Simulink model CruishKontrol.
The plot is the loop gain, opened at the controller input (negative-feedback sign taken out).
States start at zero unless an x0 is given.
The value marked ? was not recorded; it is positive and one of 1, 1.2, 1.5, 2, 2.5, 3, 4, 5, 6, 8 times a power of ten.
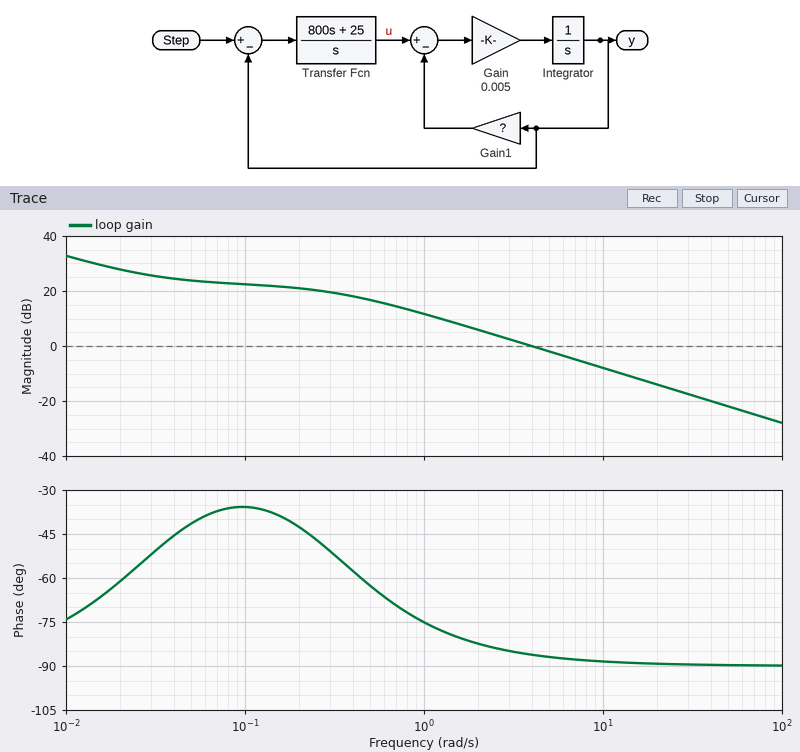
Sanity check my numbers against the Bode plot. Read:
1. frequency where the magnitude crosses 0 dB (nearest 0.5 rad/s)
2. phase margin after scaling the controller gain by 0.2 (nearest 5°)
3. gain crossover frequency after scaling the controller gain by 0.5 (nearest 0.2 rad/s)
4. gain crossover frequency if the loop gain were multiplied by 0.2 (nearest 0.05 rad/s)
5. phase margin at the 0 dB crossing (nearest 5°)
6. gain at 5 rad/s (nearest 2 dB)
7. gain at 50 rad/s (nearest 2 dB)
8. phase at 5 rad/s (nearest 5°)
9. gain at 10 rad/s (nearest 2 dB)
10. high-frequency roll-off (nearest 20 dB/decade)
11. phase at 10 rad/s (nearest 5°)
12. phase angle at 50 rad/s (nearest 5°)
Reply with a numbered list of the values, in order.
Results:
1. 4.0 rad/s
2. 110°
3. 2.0 rad/s
4. 0.75 rad/s
5. 95°
6. -2 dB
7. -22 dB
8. -85°
9. -8 dB
10. -20 dB/decade
11. -90°
12. -90°
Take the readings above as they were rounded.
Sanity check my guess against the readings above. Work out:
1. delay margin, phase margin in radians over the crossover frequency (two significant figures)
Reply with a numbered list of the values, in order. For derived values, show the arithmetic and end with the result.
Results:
1. 95 × π / 180 / 4 = 0.41 s
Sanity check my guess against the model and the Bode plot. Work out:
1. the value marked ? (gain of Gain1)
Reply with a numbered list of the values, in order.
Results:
1. 60
